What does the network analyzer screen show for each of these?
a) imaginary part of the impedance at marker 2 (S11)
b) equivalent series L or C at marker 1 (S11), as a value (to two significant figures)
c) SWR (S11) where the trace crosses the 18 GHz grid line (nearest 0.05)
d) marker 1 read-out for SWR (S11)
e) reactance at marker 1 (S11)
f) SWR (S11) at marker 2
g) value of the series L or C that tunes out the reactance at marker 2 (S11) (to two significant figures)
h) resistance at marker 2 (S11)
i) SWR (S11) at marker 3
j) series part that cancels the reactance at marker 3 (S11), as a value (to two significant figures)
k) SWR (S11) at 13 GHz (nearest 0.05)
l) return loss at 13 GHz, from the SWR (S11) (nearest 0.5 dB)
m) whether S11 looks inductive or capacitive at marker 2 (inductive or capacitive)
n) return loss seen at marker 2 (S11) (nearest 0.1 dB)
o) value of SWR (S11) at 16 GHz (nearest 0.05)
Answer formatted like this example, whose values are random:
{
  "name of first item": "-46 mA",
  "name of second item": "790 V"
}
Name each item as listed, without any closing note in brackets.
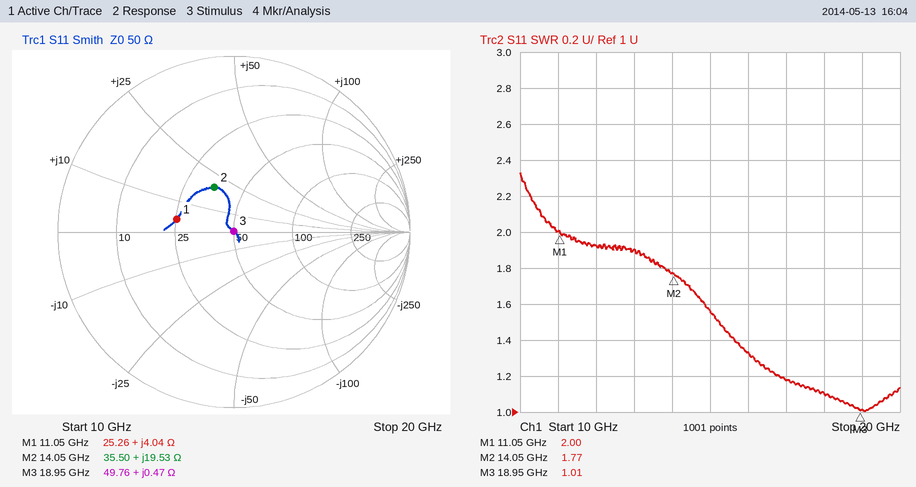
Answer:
{
  "imaginary part of the impedance at marker 2": "+19.53 Ω",
  "equivalent series L or C at marker 1 (S11), as a value": "58 pH",
  "SWR (S11) where the trace crosses the 18 GHz grid line": "1.10",
  "marker 1 read-out for SWR": "2.00",
  "reactance at marker 1": "+4.04 Ω",
  "SWR (S11) at marker 2": "1.77",
  "value of the series L or C that tunes out the reactance at marker 2 (S11)": "580 fF",
  "resistance at marker 2": "35.50 Ω",
  "SWR (S11) at marker 3": "1.01",
  "series part that cancels the reactance at marker 3 (S11), as a value": "18 pF",
  "SWR (S11) at 13 GHz": "1.90",
  "return loss at 13 GHz, from the SWR (S11)": "10.0 dB",
  "whether S11 looks inductive or capacitive at marker 2": "inductive",
  "return loss seen at marker 2 (S11)": "11.1 dB",
  "value of SWR (S11) at 16 GHz": "1.35"
}
